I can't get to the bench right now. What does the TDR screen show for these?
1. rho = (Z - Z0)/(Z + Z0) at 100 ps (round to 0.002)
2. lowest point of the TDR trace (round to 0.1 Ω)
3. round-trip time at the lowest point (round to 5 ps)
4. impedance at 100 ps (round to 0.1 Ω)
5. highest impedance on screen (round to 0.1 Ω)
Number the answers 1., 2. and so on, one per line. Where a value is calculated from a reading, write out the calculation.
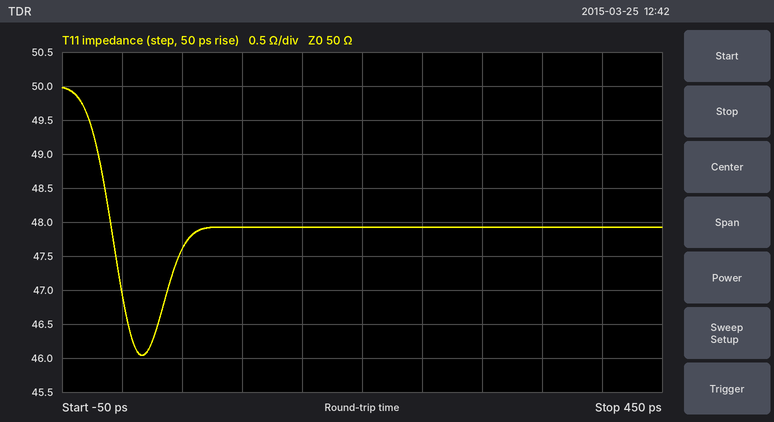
1. (47.9 − 50)/(47.9 + 50) ≈ -0.022
2. 46.0 Ω
3. 15 ps
4. 47.9 Ω
5. 50.0 Ω
